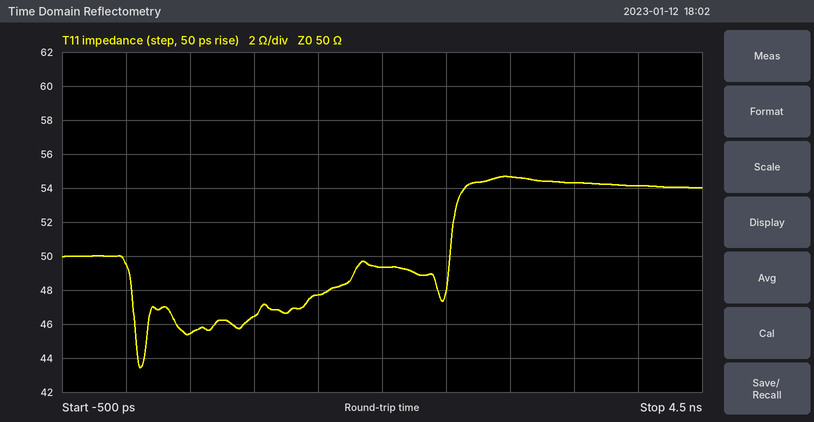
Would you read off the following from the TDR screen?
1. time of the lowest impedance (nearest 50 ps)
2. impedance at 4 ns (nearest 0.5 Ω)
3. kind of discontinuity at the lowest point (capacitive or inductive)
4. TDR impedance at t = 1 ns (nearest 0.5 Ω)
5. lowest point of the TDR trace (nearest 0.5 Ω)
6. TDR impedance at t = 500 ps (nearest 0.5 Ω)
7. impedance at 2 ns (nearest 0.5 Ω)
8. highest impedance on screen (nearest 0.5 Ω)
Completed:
100 ps
54.0 Ω
capacitive
46.5 Ω
43.5 Ω
45.5 Ω
49.5 Ω
54.5 Ω
